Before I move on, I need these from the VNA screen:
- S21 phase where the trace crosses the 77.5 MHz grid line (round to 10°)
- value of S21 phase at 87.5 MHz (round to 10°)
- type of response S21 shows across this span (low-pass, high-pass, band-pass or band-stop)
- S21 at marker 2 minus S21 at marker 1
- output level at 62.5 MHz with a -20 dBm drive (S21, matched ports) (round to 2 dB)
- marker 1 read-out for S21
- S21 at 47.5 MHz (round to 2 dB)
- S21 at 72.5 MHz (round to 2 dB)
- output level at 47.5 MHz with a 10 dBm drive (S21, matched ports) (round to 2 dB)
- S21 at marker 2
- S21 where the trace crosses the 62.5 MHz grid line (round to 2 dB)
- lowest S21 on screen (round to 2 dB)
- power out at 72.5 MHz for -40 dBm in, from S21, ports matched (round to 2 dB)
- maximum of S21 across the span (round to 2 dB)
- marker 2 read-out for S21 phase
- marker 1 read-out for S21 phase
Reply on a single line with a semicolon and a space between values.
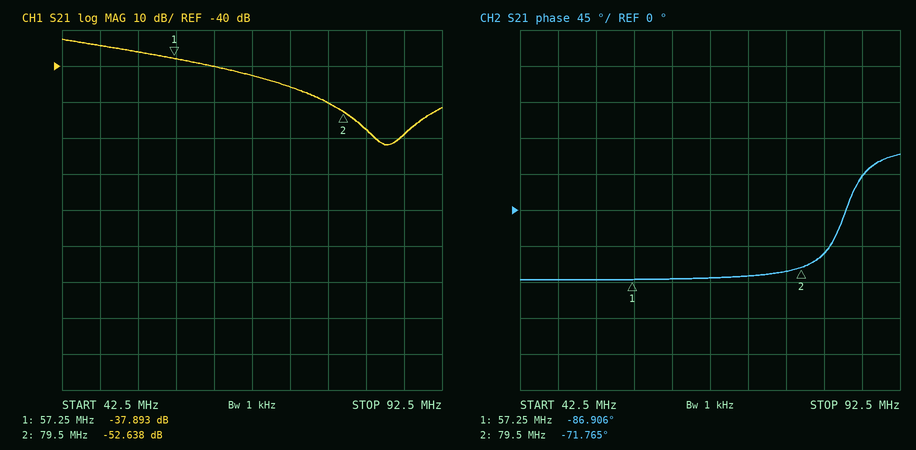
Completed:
-80°; 40°; low-pass; -14.745 dB; -60 dBm; -37.893 dB; -34 dB; -46 dB; -24 dBm; -52.638 dB; -40 dB; -62 dB; -86 dBm; -32 dB; -71.765°; -86.906°
